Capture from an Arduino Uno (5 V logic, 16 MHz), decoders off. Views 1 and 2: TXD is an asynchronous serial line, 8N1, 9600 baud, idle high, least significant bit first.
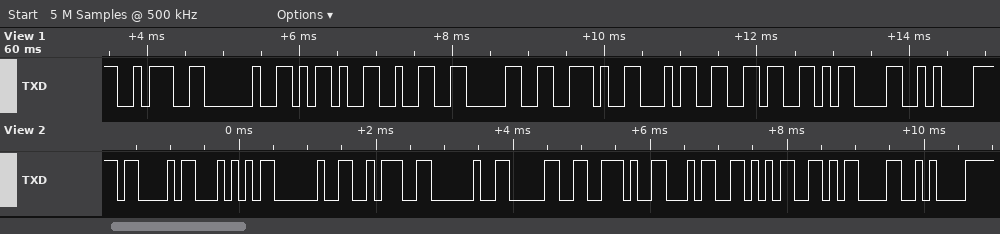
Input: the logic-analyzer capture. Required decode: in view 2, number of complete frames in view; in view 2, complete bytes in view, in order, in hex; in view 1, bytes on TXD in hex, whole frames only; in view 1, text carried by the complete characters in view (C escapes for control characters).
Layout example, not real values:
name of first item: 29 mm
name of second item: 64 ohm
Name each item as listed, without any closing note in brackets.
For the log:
in view 2, number of complete frames in view: 11
in view 2, complete bytes in view, in order, in hex: 0x43 0x54 0x20 0x3A 0x20 0x30 0x2E 0x34 0x35 0x0D 0x0A
in view 1, bytes on TXD in hex, whole frames only: 3A 20 2D 32 30 2E 34 36 0D 0A
in view 1, text carried by the complete characters in view: ": -20.46\r\n"
